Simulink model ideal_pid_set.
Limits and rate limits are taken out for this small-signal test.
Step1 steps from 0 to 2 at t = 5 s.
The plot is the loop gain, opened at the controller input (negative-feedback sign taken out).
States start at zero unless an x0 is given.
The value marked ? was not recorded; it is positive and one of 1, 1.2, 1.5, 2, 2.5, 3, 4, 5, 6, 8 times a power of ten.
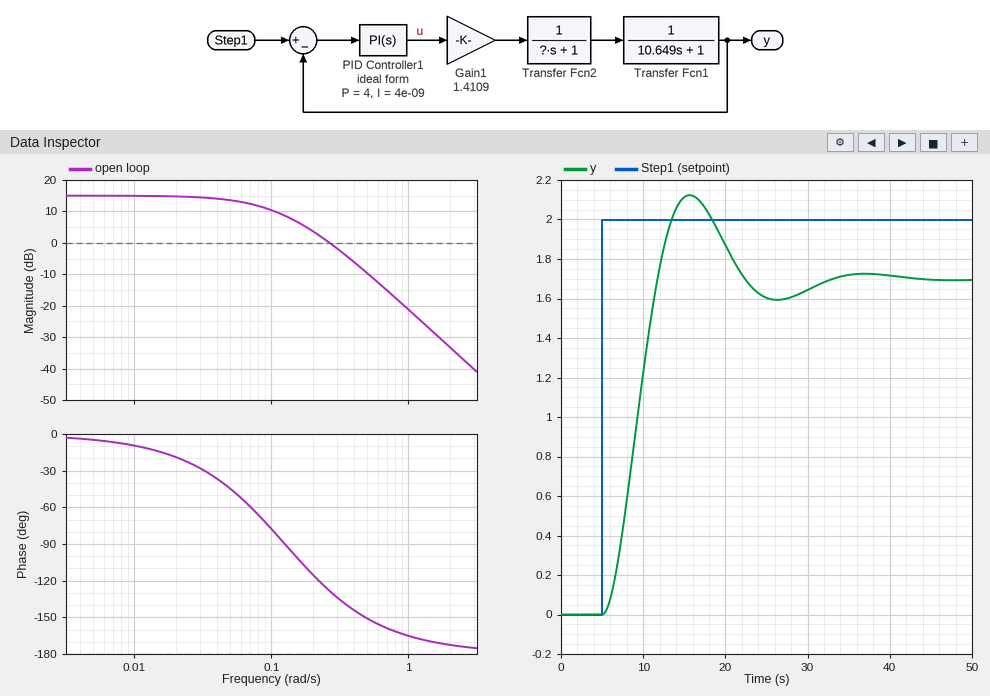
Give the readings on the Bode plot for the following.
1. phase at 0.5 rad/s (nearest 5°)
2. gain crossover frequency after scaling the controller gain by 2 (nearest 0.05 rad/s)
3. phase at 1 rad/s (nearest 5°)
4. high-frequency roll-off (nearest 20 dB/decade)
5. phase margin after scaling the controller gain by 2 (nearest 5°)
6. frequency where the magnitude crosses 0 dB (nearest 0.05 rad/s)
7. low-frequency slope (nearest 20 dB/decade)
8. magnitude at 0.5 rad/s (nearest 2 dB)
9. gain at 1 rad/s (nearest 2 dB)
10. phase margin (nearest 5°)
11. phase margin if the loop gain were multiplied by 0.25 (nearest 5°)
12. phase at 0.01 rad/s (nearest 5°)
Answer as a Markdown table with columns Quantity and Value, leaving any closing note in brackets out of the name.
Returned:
| Quantity | Value |
|---|---|
| phase at 0.5 rad/s | -150° |
| gain crossover frequency after scaling the controller gain by 2 | 0.40 rad/s |
| phase at 1 rad/s | -165° |
| high-frequency roll-off | -40 dB/decade |
| phase margin after scaling the controller gain by 2 | 35° |
| frequency where the magnitude crosses 0 dB | 0.25 rad/s |
| low-frequency slope | 0 dB/decade |
| magnitude at 0.5 rad/s | -10 dB |
| gain at 1 rad/s | -22 dB |
| phase margin | 50° |
| phase margin if the loop gain were multiplied by 0.25 | 115° |
| phase at 0.01 rad/s | -10° |
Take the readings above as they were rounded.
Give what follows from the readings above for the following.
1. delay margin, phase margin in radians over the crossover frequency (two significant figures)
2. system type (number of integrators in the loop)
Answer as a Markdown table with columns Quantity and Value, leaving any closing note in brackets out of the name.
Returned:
| Quantity | Value |
|---|---|
| delay margin, phase margin in radians over the crossover frequency | 3.5 s |
| system type | 0 |
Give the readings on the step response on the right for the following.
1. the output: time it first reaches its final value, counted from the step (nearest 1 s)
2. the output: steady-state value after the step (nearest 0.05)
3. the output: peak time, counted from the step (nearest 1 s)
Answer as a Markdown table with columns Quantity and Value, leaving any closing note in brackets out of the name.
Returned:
| Quantity | Value |
|---|---|
| the output: time it first reaches its final value, counted from the step | 7 s |
| the output: steady-state value after the step | 1.70 |
| the output: peak time, counted from the step | 11 s |
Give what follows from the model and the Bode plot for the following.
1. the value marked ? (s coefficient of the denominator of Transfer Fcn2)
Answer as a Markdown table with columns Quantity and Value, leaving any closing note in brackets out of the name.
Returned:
| Quantity | Value |
|---|---|
| the value marked ? | 6 |
